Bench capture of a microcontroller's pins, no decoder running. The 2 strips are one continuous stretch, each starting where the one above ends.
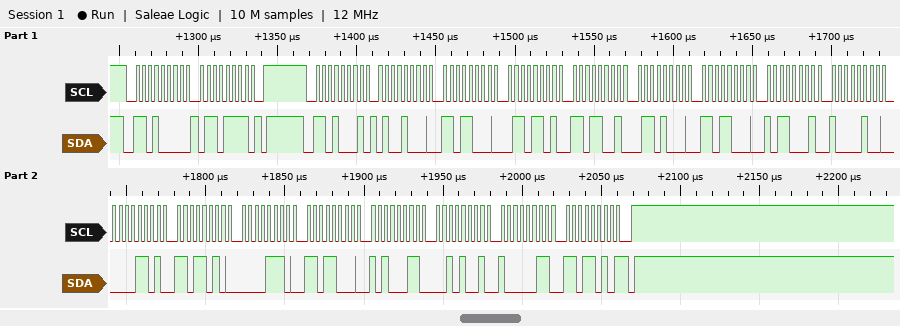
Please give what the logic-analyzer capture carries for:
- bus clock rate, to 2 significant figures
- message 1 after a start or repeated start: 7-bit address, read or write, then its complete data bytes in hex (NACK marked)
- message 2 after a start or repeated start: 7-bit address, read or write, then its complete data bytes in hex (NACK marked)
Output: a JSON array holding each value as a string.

["250 kHz", "0x68 write: 6F", "0x68 read: 48 D8 6D D9 68 D8 B1 84 0D DA 0E D8 A3 29 83 DA NACK"]
